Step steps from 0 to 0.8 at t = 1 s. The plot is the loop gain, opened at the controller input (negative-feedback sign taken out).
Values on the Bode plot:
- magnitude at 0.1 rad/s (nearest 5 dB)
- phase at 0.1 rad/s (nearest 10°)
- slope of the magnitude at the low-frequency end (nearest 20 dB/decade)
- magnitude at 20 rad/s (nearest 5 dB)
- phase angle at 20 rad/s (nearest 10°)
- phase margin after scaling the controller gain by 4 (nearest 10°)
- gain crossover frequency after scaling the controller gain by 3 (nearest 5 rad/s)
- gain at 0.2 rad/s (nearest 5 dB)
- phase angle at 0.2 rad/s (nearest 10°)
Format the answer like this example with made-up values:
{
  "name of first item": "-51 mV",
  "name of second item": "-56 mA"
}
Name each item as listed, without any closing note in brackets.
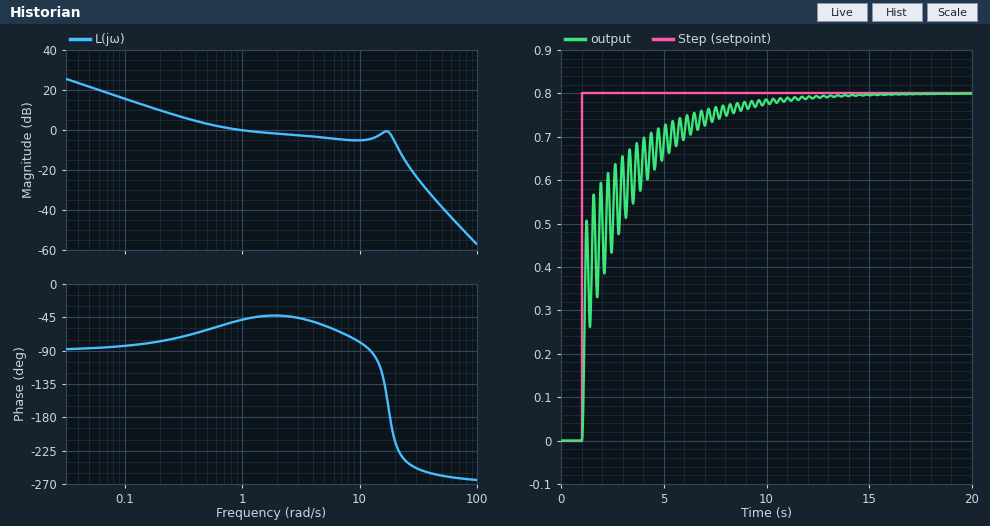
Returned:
{
  "magnitude at 0.1 rad/s": "15 dB",
  "phase at 0.1 rad/s": "-80°",
  "slope of the magnitude at the low-frequency end": "-20 dB/decade",
  "magnitude at 20 rad/s": "-5 dB",
  "phase angle at 20 rad/s": "-210°",
  "phase margin after scaling the controller gain by 4": "-50°",
  "gain crossover frequency after scaling the controller gain by 3": "20 rad/s",
  "gain at 0.2 rad/s": "10 dB",
  "phase angle at 0.2 rad/s": "-80°"
}
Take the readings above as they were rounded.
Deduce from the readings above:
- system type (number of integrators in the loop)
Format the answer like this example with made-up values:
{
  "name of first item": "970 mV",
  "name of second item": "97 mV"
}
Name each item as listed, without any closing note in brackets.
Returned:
{
  "system type": "1"
}
